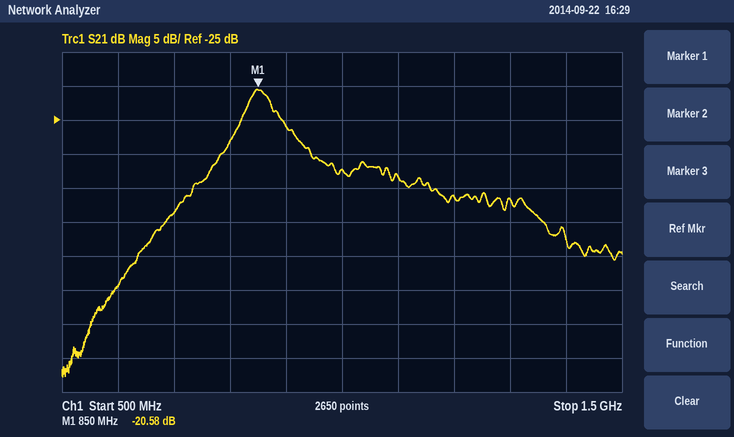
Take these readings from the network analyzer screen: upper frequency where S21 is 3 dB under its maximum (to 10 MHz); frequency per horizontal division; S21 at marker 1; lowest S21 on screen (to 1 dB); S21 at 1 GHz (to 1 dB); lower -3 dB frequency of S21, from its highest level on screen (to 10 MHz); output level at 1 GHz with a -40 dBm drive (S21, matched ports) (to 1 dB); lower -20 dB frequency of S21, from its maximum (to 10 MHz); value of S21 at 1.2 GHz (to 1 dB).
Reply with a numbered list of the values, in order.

1. 880 MHz
2. 100 MHz
3. -20.58 dB
4. -63 dB
5. -32 dB
6. 830 MHz
7. -72 dBm
8. 680 MHz
9. -36 dB
